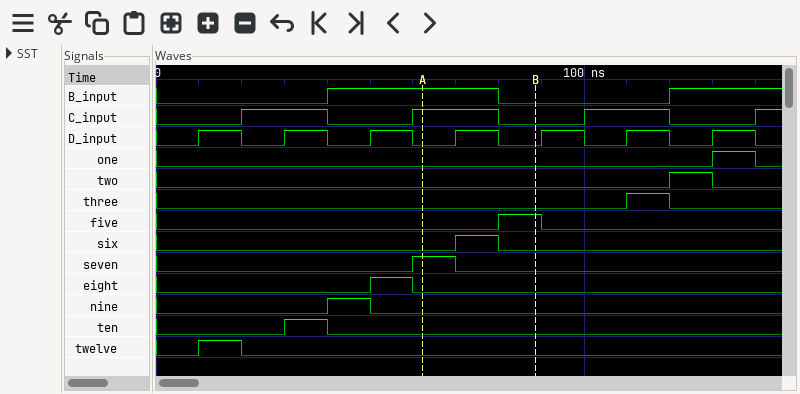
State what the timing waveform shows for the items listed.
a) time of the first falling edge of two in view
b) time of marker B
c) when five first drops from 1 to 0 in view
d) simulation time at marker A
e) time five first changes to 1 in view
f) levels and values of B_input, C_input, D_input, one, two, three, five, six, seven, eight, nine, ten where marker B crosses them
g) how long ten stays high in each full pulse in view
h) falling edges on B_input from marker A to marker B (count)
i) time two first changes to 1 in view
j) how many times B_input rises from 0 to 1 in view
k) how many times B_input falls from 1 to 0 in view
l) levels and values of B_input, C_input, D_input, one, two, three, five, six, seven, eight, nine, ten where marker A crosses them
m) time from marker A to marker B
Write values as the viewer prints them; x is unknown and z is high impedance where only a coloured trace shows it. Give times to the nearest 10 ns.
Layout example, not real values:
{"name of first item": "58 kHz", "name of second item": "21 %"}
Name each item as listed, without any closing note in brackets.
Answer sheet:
{"time of the first falling edge of two in view": "130 ns", "time of marker B": "90 ns", "when five first drops from 1 to 0 in view": "90 ns", "simulation time at marker A": "60 ns", "time five first changes to 1 in view": "80 ns", "levels and values of B_input, C_input, D_input, one, two, three, five, six, seven, eight, nine, ten where marker B crosses them": "B_input=0, C_input=0, D_input=0, one=0, two=0, three=0, five=1, six=0, seven=0, eight=0, nine=0, ten=0", "how long ten stays high in each full pulse in view": "10 ns", "falling edges on B_input from marker A to marker B": "1", "time two first changes to 1 in view": "120 ns", "how many times B_input rises from 0 to 1 in view": "2", "how many times B_input falls from 1 to 0 in view": "1", "levels and values of B_input, C_input, D_input, one, two, three, five, six, seven, eight, nine, ten where marker A crosses them": "B_input=1, C_input=1, D_input=0, one=0, two=0, three=0, five=0, six=0, seven=1, eight=0, nine=0, ten=0", "time from marker A to marker B": "30 ns"}
